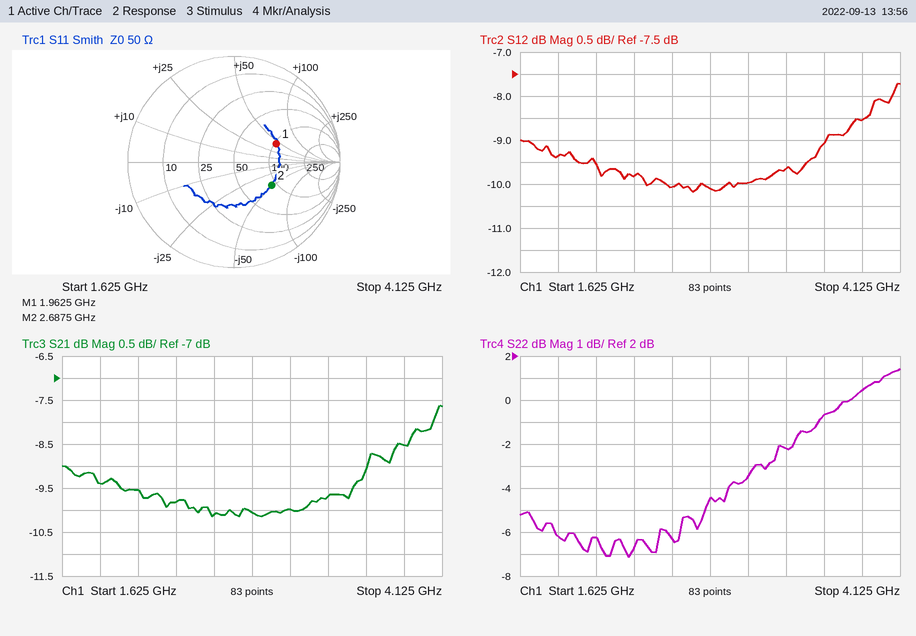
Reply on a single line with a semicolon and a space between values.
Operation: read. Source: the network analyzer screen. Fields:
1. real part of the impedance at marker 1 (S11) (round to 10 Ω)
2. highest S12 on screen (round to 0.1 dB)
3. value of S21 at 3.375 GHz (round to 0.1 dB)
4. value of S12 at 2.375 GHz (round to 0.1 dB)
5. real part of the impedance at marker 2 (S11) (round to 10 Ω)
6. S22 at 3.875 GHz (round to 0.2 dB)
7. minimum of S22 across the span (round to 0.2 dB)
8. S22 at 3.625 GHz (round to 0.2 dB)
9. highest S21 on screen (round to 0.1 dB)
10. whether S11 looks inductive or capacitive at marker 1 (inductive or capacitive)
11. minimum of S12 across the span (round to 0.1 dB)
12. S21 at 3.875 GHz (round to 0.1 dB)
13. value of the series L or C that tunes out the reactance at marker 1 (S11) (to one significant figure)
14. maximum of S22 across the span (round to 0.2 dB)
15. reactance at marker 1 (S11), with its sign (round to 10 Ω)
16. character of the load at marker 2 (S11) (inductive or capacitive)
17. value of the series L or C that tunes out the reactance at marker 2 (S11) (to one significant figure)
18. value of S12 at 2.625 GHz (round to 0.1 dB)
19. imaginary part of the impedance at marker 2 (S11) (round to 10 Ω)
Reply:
100 Ω; -7.7 dB; -9.7 dB; -9.8 dB; 90 Ω; 0.4 dB; -7.2 dB; -0.6 dB; -7.6 dB; inductive; -10.2 dB; -8.5 dB; 2 pF; 1.4 dB; +40 Ω; capacitive; 3 nH; -10.1 dB; -50 Ω
